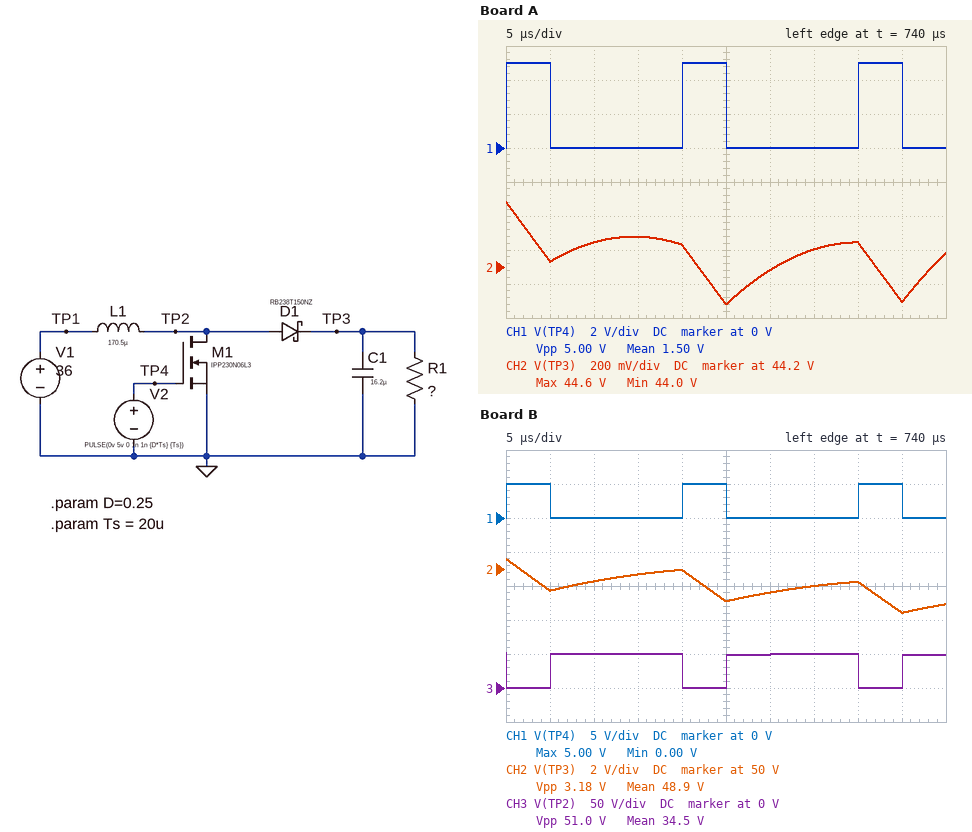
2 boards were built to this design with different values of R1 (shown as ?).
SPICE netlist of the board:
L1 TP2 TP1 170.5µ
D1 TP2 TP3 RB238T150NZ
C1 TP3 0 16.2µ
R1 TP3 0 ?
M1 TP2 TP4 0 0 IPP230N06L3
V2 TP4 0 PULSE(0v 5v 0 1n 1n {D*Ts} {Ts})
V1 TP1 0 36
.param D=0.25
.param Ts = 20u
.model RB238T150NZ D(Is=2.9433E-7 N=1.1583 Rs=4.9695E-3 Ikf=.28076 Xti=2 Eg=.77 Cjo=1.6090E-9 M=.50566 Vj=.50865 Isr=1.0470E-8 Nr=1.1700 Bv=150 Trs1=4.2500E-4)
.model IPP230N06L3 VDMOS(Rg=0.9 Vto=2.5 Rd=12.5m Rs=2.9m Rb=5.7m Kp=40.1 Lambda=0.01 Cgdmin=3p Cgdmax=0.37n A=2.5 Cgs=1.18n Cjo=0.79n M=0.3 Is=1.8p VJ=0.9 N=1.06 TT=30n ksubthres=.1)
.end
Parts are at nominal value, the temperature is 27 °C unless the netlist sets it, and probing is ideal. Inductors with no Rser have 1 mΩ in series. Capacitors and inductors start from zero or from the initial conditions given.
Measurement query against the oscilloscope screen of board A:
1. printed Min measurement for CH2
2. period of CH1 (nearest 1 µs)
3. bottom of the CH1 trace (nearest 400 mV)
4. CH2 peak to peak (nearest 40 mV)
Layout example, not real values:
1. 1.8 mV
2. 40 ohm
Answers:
1. 44.0 V
2. 20 µs
3. 0 V
4. 600 mV
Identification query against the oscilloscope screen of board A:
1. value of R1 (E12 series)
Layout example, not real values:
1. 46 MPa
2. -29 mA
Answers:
1. 39 Ω
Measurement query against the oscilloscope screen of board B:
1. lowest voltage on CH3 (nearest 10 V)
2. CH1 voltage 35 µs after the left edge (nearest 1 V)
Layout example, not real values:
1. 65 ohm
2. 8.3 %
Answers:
1. 0 V
2. 0 V
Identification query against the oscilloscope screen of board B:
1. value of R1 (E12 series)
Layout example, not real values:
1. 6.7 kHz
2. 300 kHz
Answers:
1. 8.2 Ω
